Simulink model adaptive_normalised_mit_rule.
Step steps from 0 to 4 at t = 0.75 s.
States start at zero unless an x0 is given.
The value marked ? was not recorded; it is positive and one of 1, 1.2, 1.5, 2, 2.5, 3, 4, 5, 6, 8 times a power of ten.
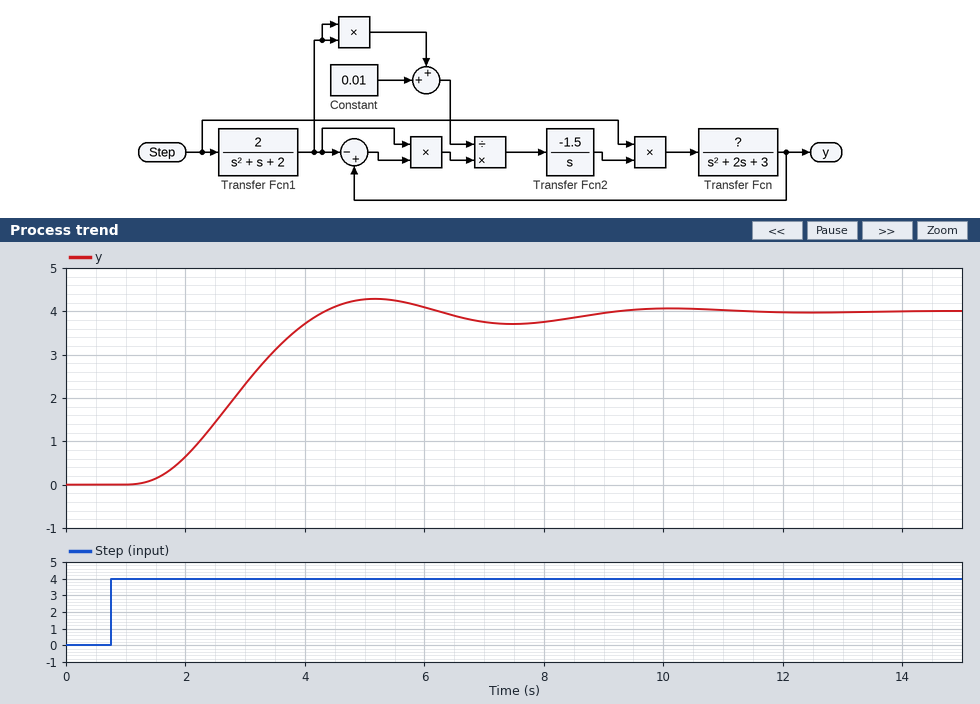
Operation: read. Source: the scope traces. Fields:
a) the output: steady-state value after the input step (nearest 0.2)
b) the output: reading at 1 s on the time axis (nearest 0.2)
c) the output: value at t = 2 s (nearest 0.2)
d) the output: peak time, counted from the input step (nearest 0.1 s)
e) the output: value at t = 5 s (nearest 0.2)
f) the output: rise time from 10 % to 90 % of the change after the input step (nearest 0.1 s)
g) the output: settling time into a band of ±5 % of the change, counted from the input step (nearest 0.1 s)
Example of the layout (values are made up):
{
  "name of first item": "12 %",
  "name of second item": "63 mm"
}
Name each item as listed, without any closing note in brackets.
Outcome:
{
  "the output: steady-state value after the input step": "4.0",
  "the output: reading at 1 s on the time axis": "0.0",
  "the output: value at t = 2 s": "0.6",
  "the output: peak time, counted from the input step": "4.4 s",
  "the output: value at t = 5 s": "4.2",
  "the output: rise time from 10 % to 90 % of the change after the input step": "2.1 s",
  "the output: settling time into a band of ±5 % of the change, counted from the input step": "7.5 s"
}
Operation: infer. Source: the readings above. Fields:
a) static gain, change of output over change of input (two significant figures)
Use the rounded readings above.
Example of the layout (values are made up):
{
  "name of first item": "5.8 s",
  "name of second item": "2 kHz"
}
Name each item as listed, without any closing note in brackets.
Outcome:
{
  "static gain, change of output over change of input": "1.0"
}
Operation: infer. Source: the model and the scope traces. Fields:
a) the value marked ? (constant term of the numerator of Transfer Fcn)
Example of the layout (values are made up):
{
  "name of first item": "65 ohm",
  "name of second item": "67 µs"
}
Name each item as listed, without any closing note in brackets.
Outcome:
{
  "the value marked ?": "1"
}
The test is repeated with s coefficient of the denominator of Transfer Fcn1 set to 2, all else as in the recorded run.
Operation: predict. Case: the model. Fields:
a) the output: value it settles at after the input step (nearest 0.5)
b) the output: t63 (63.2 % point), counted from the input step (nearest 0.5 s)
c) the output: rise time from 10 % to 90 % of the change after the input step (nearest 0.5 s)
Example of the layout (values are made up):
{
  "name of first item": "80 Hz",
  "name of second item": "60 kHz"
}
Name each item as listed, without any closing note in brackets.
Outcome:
{
  "the output: value it settles at after the input step": "4.0",
  "the output: t63 (63.2 % point), counted from the input step": "2.5 s",
  "the output: rise time from 10 % to 90 % of the change after the input step": "2.5 s"
}
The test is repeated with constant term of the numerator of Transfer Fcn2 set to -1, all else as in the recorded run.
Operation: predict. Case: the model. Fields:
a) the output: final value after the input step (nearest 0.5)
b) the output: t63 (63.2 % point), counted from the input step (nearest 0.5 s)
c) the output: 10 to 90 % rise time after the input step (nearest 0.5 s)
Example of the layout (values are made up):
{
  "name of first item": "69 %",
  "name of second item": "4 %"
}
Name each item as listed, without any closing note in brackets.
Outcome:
{
  "the output: final value after the input step": "4.0",
  "the output: t63 (63.2 % point), counted from the input step": "3.0 s",
  "the output: 10 to 90 % rise time after the input step": "5.5 s"
}
